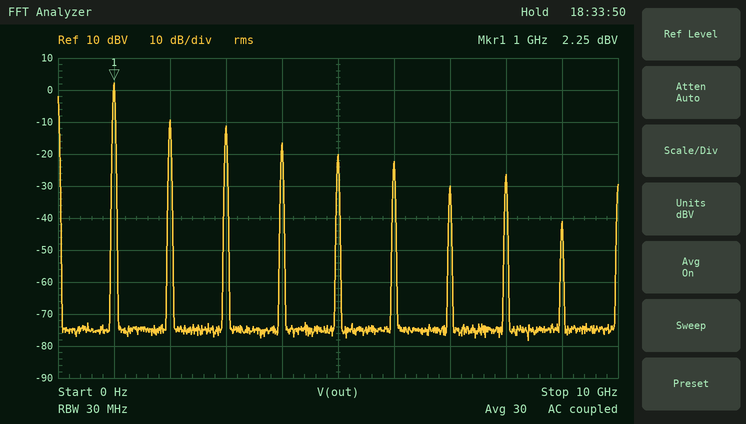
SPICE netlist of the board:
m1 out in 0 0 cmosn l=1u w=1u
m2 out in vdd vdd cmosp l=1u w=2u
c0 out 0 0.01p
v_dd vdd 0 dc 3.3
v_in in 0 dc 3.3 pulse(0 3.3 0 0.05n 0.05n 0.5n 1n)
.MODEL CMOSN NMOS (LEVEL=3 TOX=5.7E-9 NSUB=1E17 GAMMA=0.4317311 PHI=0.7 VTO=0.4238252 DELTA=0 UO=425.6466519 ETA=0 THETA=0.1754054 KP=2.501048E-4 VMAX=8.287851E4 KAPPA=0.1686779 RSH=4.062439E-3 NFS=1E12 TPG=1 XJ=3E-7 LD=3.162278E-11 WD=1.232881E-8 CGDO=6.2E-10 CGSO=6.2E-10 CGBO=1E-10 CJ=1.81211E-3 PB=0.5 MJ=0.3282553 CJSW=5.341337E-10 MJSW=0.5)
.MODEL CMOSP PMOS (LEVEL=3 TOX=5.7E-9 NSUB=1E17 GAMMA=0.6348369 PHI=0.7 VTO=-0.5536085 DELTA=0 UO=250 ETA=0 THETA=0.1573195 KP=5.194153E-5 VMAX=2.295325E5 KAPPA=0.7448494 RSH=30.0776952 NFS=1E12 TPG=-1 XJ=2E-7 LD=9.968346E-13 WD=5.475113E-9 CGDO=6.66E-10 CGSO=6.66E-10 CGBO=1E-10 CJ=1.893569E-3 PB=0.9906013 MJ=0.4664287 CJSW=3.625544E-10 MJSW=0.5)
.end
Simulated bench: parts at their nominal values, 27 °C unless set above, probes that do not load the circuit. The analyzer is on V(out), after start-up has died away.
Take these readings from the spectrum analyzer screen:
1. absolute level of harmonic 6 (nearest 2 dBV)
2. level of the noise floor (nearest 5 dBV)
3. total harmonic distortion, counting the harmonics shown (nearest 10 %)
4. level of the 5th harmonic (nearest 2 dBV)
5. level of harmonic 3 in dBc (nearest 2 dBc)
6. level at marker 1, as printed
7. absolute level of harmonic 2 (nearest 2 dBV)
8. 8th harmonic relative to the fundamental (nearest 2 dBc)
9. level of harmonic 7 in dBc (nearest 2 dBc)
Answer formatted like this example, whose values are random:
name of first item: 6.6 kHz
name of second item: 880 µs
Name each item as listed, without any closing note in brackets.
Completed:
absolute level of harmonic 6: -22 dBV
level of the noise floor: -75 dBV
total harmonic distortion, counting the harmonics shown: 40 %
level of the 5th harmonic: -20 dBV
level of harmonic 3 in dBc: -14 dBc
level at marker 1, as printed: 2.25 dBV
absolute level of harmonic 2: -10 dBV
8th harmonic relative to the fundamental: -28 dBc
level of harmonic 7 in dBc: -32 dBc
